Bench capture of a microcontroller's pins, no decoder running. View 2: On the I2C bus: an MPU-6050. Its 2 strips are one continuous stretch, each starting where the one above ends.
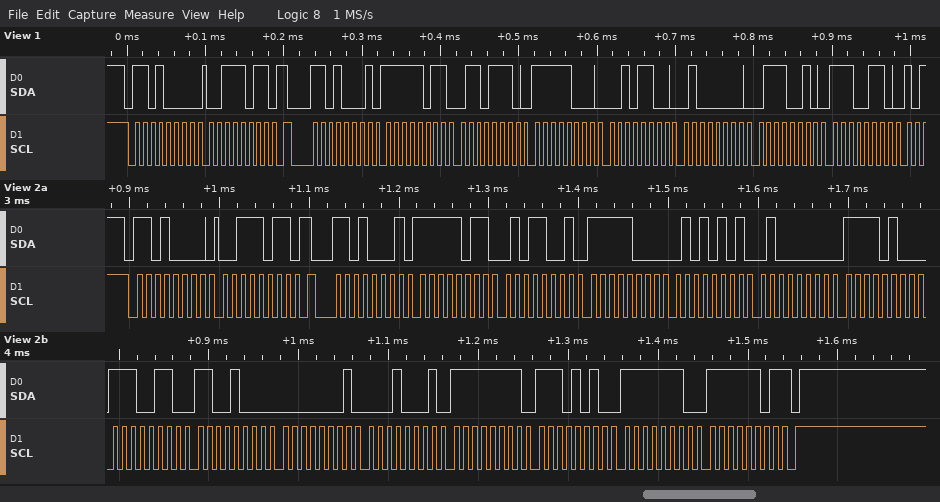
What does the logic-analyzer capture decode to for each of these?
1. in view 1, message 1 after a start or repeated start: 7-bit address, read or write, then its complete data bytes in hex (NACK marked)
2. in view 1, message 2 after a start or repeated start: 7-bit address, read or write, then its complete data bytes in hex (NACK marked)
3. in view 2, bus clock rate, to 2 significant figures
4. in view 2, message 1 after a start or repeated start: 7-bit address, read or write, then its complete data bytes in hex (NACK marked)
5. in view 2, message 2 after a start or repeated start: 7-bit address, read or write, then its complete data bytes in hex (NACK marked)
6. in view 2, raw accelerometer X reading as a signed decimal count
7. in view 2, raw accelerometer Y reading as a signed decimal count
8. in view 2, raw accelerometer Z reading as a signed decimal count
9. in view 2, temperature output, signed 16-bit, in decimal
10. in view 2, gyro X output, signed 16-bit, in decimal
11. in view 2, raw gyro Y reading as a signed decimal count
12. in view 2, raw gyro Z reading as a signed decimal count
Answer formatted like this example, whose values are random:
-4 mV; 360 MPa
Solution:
0x68 write: 3B; 0x68 read: FB 6E F8 2C 40 72 E6; 100 kHz; 0x68 write: 3B; 0x68 read: FB 59 F8 55 40 F4 E6 C8 01 11 FF EA FE FD NACK; -1191; -1963; 16628; -6456; 273; -22; -259
